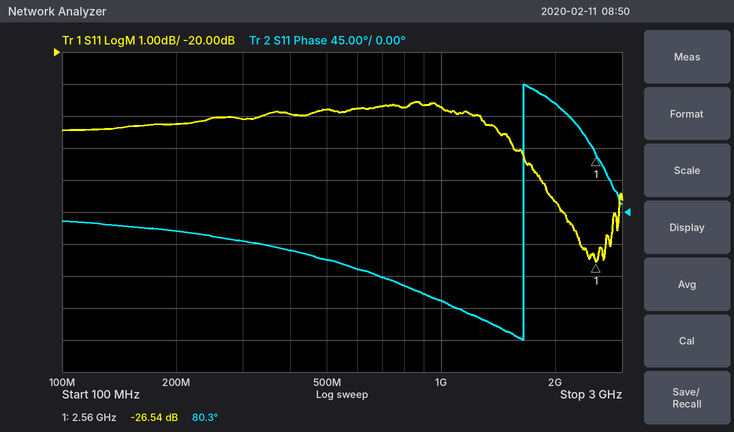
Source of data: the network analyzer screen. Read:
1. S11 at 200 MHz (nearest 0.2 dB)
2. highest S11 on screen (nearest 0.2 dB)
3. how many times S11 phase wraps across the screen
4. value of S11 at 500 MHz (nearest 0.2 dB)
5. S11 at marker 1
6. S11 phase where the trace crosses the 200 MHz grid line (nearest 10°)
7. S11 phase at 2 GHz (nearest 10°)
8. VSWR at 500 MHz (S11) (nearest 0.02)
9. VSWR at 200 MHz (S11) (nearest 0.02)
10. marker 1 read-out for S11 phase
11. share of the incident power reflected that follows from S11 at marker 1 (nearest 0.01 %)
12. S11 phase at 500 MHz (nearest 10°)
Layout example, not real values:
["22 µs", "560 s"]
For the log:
["-22.2 dB", "-21.6 dB", "1", "-21.8 dB", "-26.54 dB", "-30°", "150°", "1.18", "1.16", "80.3°", "0.22 %", "-70°"]
